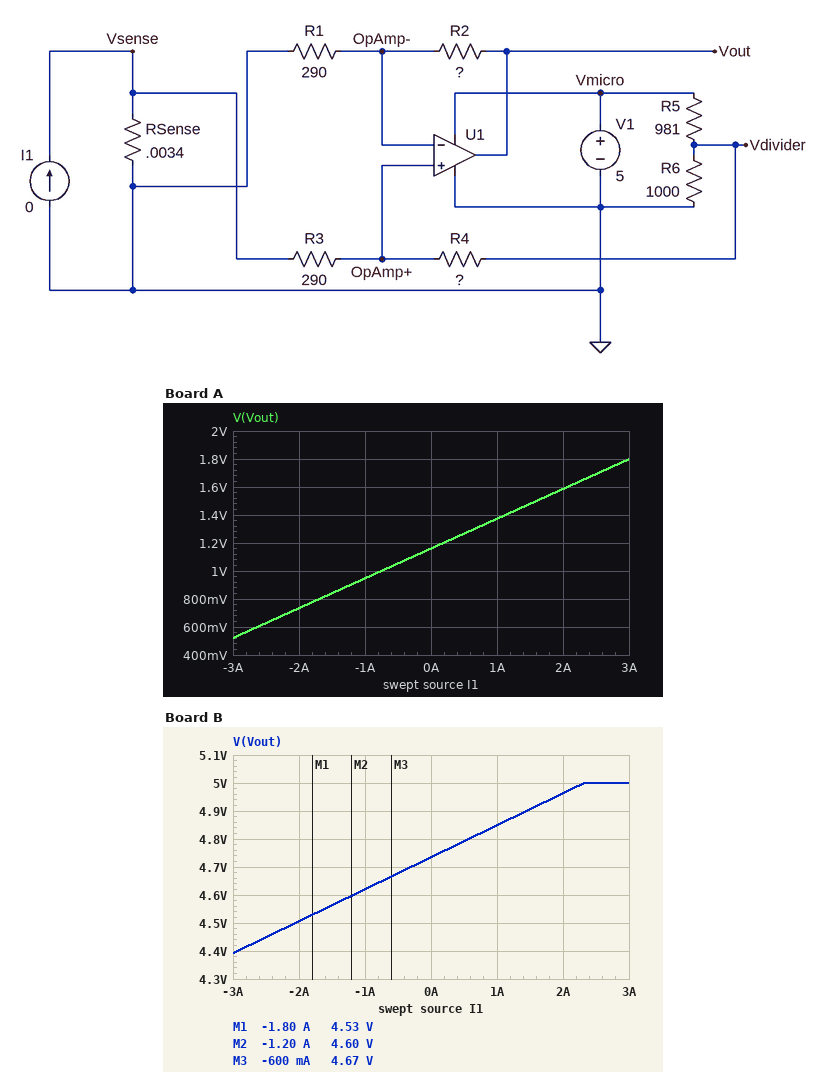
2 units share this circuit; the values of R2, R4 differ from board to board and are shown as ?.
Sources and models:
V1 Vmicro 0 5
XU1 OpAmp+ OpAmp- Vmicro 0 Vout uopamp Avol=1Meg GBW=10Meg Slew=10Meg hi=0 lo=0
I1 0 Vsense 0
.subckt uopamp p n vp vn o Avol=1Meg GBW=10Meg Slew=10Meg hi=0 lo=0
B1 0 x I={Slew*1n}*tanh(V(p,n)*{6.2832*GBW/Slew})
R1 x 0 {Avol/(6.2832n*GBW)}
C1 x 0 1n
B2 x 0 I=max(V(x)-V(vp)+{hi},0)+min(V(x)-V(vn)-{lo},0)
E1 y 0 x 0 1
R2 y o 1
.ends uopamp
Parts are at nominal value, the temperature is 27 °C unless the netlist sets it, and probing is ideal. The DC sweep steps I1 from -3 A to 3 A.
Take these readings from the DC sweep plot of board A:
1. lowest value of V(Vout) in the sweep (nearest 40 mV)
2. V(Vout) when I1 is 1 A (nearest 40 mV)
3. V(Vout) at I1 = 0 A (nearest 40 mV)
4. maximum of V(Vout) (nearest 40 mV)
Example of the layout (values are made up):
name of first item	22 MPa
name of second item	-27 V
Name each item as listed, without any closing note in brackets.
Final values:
lowest value of V(Vout) in the sweep	520 mV
V(Vout) when I1 is 1 A	1.36 V
V(Vout) at I1 = 0 A	1.16 V
maximum of V(Vout)	1.80 V
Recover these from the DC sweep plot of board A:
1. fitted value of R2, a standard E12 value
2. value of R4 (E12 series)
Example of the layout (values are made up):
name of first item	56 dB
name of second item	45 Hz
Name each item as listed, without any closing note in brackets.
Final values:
fitted value of R2, a standard E12 value	18 kΩ
value of R4	39 kΩ
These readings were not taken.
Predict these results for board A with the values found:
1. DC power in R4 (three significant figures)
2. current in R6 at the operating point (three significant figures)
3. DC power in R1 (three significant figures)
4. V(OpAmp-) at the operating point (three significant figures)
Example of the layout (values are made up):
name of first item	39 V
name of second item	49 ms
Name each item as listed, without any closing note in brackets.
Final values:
DC power in R4	157 µW
current in R6 at the operating point	2.49 mA
DC power in R1	1.17 µW
V(OpAmp-) at the operating point	18.4 mV
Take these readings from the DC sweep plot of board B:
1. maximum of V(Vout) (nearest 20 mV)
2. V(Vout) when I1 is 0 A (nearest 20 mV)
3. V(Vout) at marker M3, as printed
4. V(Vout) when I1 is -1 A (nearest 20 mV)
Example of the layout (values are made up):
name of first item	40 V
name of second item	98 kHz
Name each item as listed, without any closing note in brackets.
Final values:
maximum of V(Vout)	5.00 V
V(Vout) when I1 is 0 A	4.74 V
V(Vout) at marker M3, as printed	4.67 V
V(Vout) when I1 is -1 A	4.62 V
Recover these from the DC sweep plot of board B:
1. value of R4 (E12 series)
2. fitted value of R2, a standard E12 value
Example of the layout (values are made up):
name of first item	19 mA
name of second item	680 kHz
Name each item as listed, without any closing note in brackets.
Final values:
value of R4	4.7 kΩ
fitted value of R2, a standard E12 value	10 kΩ
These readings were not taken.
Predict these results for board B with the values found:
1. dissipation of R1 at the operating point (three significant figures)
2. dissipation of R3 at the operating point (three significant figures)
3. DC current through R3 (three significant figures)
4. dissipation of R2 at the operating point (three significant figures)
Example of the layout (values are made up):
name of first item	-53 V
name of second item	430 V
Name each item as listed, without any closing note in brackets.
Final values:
dissipation of R1 at the operating point	61.4 µW
dissipation of R3 at the operating point	61.4 µW
DC current through R3	460 µA
dissipation of R2 at the operating point	2.12 mW
